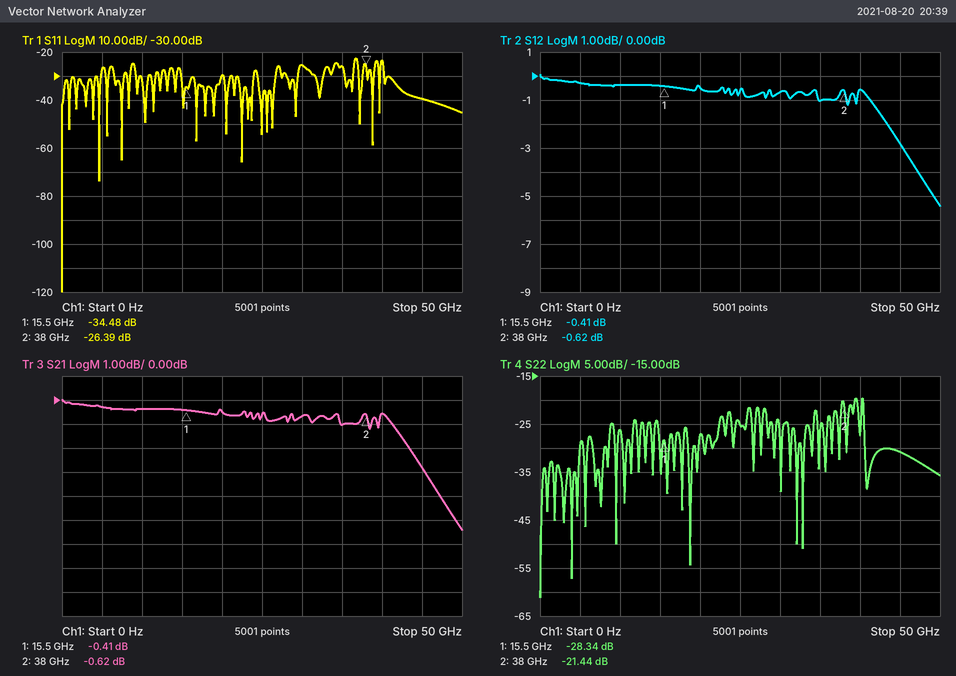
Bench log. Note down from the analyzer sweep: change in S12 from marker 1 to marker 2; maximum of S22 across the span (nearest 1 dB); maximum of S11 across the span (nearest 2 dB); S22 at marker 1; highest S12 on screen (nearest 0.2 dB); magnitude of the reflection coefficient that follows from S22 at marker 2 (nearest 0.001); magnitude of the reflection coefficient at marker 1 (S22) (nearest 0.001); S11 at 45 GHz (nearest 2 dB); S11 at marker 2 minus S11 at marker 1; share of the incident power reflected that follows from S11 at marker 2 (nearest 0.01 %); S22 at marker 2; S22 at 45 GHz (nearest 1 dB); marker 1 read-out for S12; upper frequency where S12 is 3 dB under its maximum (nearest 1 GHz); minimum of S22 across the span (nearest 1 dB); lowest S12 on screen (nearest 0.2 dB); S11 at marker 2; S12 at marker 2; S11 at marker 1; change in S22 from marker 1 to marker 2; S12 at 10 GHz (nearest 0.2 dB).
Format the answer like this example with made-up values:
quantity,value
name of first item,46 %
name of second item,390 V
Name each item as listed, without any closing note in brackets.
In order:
quantity,value
change in S12 from marker 1 to marker 2,-0.21 dB
maximum of S22 across the span,-20 dB
maximum of S11 across the span,-22 dB
S22 at marker 1,-28.34 dB
highest S12 on screen,0.0 dB
magnitude of the reflection coefficient that follows from S22 at marker 2,0.085
magnitude of the reflection coefficient at marker 1 (S22),0.038
S11 at 45 GHz,-40 dB
S11 at marker 2 minus S11 at marker 1,8.09 dB
share of the incident power reflected that follows from S11 at marker 2,0.23 %
S22 at marker 2,-21.44 dB
S22 at 45 GHz,-31 dB
marker 1 read-out for S12,-0.41 dB
upper frequency where S12 is 3 dB under its maximum,45 GHz
minimum of S22 across the span,-61 dB
lowest S12 on screen,-5.4 dB
S11 at marker 2,-26.39 dB
S12 at marker 2,-0.62 dB
S11 at marker 1,-34.48 dB
change in S22 from marker 1 to marker 2,6.90 dB
S12 at 10 GHz,-0.4 dB
